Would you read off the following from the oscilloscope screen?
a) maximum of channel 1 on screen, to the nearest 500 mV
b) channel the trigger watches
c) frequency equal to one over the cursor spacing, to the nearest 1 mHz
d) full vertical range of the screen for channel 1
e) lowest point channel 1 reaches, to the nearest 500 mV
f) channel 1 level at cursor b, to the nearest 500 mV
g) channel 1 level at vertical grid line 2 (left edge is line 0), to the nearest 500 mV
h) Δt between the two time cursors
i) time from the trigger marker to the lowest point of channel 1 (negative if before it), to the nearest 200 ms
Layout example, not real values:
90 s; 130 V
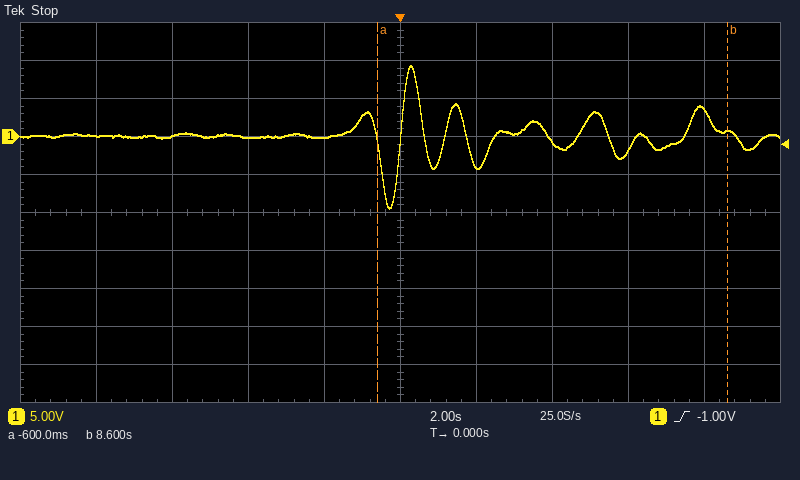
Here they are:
9.5 V; channel 1; 109 mHz; 50 V; -9.5 V; 500 mV; 0.0 V; 9.2 s; -200 ms
